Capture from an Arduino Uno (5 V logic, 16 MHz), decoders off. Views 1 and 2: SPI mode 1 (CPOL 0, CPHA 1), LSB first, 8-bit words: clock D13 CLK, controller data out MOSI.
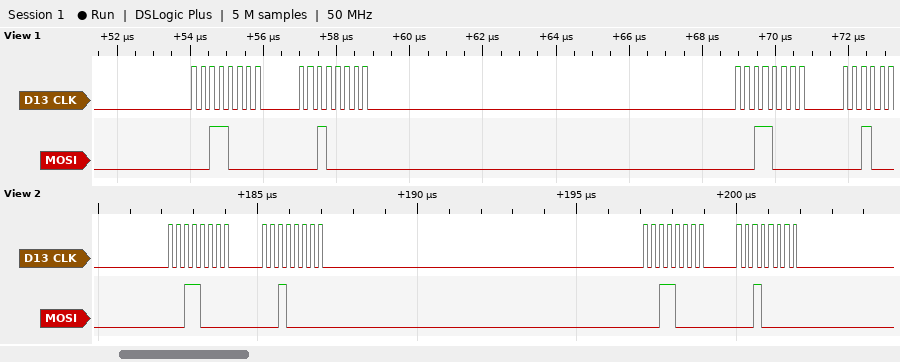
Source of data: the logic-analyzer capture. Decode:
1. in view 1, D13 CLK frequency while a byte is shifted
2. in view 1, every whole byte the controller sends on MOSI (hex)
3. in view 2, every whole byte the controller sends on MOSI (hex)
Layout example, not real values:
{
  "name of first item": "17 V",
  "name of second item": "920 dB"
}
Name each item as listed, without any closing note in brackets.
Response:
{
  "in view 1, D13 CLK frequency while a byte is shifted": "4 MHz",
  "in view 1, every whole byte the controller sends on MOSI": "0C 04 0C",
  "in view 2, every whole byte the controller sends on MOSI": "0x0C 0x04 0x0C 0x04"
}
